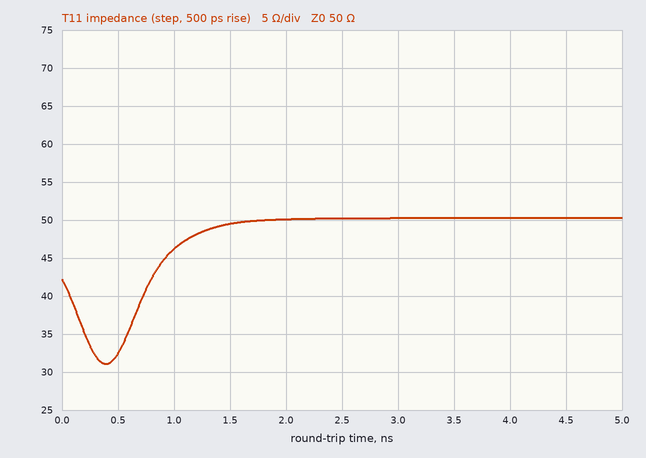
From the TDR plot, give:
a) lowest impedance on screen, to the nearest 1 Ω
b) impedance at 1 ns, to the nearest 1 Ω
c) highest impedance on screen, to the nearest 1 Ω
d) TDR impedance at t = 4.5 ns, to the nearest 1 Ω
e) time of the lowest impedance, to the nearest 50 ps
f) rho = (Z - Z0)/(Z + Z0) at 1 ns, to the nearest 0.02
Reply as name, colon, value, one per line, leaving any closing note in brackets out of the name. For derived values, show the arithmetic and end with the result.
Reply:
lowest impedance on screen, to the nearest 1 Ω: 31 Ω
impedance at 1 ns, to the nearest 1 Ω: 46 Ω
highest impedance on screen, to the nearest 1 Ω: 50 Ω
TDR impedance at t = 4.5 ns, to the nearest 1 Ω: 50 Ω
time of the lowest impedance, to the nearest 50 ps: 400 ps
rho = (Z - Z0)/(Z + Z0) at 1 ns, to the nearest 0.02: (46 − 50)/(46 + 50) ≈ -0.04
